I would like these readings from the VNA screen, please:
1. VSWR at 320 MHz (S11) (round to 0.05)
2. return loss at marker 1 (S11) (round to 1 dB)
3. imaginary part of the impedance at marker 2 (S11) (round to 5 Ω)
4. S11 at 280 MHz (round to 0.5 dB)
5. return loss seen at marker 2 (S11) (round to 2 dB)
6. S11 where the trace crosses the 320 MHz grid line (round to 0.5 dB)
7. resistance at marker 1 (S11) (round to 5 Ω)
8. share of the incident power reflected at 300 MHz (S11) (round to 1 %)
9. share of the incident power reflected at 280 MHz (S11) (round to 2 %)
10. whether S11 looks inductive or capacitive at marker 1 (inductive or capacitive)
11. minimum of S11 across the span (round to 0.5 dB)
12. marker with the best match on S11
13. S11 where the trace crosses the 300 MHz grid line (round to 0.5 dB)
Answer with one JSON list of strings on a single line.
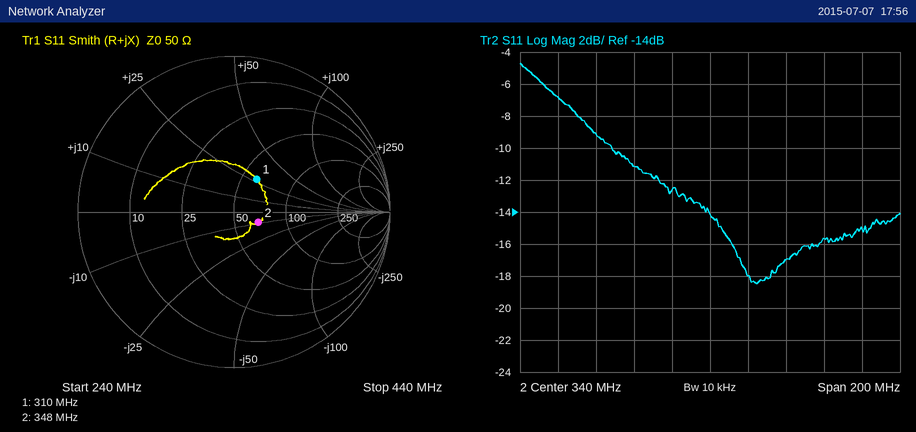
["1.60", "12 dB", "-10 Ω", "-9.0 dB", "16 dB", "-12.5 dB", "60 Ω", "8 %", "12 %", "inductive", "-18.5 dB", "marker 2", "-11.0 dB"]
